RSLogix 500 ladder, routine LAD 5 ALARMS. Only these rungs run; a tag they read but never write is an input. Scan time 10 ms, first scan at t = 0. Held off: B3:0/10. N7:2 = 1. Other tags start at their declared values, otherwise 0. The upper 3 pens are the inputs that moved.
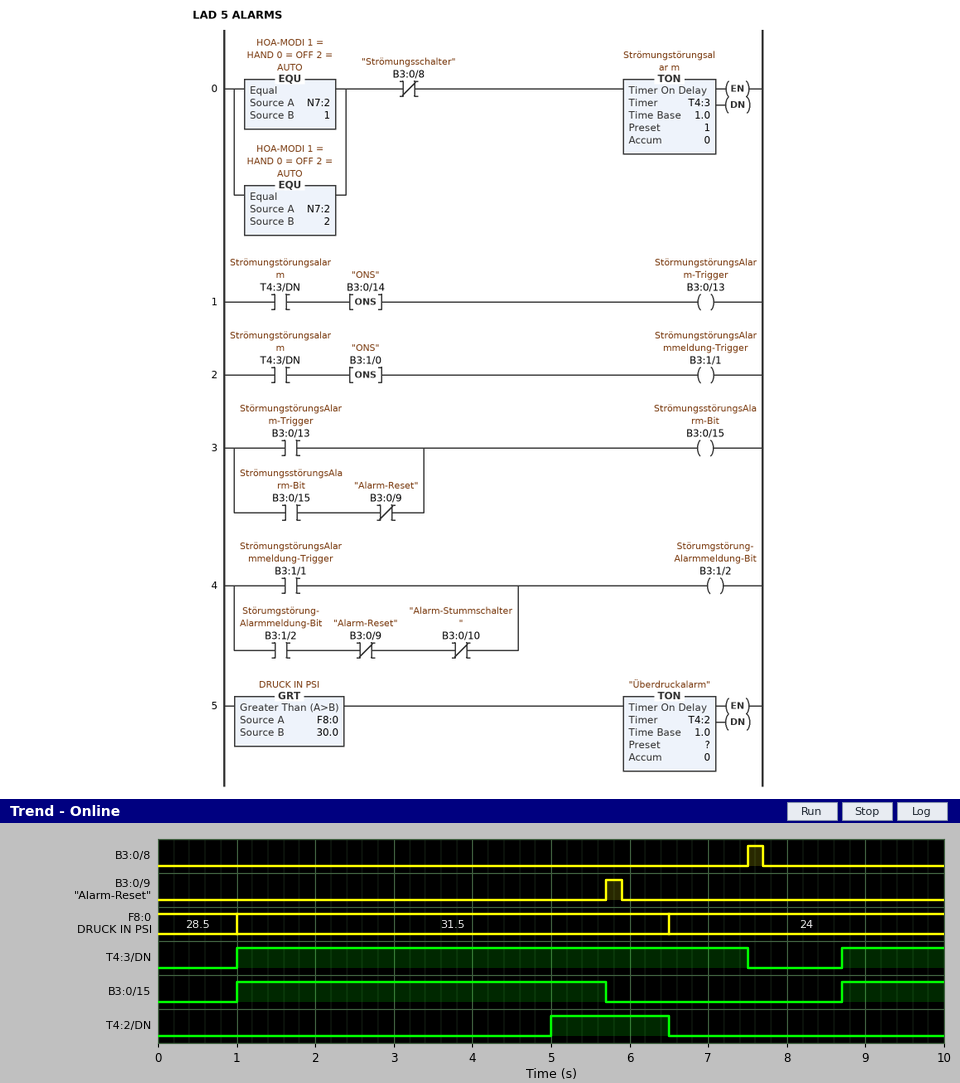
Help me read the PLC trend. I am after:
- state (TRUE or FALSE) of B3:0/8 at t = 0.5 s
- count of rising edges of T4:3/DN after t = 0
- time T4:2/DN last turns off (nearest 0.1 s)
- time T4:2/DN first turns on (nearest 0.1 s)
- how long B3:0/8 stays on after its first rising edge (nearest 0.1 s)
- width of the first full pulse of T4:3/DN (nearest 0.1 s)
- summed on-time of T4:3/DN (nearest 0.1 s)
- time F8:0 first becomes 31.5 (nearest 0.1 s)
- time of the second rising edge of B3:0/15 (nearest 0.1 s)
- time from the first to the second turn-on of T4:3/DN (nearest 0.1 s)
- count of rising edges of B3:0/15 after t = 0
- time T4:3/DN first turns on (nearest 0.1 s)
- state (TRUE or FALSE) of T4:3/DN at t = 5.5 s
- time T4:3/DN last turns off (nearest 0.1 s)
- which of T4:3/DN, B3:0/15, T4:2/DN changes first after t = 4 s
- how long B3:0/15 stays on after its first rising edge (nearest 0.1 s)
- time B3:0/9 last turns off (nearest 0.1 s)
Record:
FALSE
2
6.5 s
5.0 s
0.2 s
6.5 s
7.8 s
1.0 s
8.7 s
7.7 s
2
1.0 s
TRUE
7.5 s
T4:2/DN
4.7 s
5.9 s
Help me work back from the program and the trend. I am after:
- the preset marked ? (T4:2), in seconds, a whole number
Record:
4 s
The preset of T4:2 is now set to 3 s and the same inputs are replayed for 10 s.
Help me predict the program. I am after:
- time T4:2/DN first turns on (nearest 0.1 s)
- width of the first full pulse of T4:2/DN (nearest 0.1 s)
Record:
4.0 s
2.5 s
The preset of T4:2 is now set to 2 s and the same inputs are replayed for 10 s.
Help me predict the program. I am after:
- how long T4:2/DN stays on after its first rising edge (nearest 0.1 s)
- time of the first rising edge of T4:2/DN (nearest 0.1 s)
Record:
3.5 s
3.0 s
